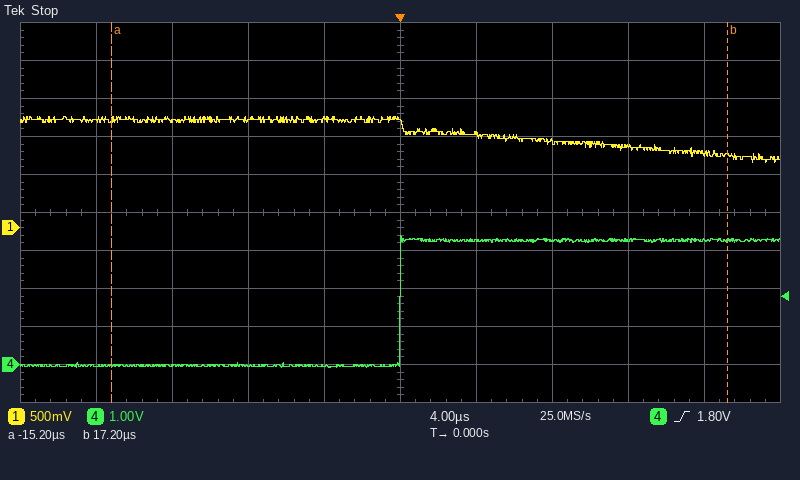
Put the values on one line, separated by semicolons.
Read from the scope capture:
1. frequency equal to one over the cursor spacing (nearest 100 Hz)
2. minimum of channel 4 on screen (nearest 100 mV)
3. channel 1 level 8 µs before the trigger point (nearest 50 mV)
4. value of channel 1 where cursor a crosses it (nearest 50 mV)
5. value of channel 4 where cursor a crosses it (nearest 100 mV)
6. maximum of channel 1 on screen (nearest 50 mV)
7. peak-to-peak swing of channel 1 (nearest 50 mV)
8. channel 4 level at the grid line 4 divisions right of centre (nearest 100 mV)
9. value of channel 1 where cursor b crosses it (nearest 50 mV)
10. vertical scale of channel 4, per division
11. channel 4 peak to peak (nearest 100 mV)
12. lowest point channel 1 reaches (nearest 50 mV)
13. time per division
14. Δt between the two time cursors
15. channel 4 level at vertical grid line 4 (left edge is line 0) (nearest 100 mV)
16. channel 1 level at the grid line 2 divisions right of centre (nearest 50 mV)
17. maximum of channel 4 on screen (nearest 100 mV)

30.9 kHz; -100 mV; 1.40 V; 1.40 V; 0.0 V; 1.45 V; 600 mV; 3.3 V; 950 mV; 1 V; 3.5 V; 850 mV; 4 µs; 32.4 µs; 0.0 V; 1.15 V; 3.4 V
